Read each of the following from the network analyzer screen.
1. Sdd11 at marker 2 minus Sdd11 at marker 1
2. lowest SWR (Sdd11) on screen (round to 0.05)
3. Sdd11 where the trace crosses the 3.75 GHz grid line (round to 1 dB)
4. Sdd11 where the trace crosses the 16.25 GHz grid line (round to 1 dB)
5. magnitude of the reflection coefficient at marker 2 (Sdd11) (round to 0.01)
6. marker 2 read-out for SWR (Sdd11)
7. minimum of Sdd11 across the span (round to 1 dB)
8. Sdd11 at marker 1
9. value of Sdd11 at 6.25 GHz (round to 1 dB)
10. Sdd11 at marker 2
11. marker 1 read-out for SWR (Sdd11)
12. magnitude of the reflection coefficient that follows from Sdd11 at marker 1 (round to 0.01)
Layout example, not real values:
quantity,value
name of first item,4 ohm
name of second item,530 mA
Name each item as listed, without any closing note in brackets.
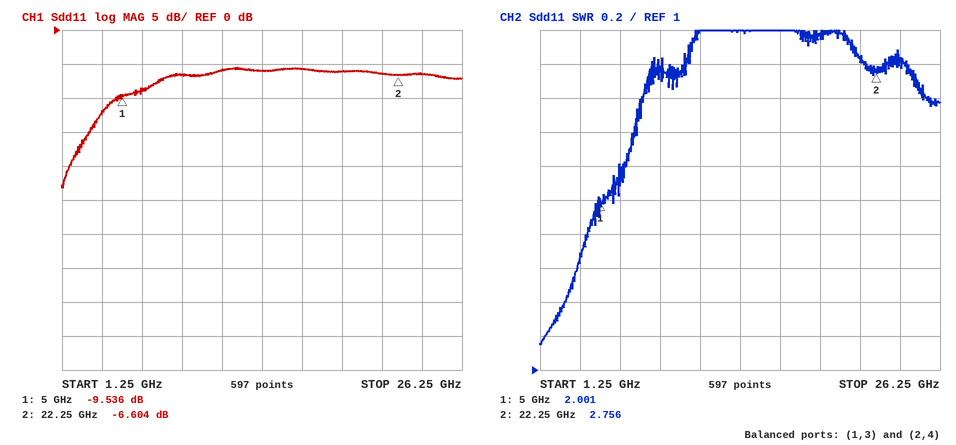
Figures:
quantity,value
Sdd11 at marker 2 minus Sdd11 at marker 1,2.932 dB
lowest SWR (Sdd11) on screen,1.15
Sdd11 where the trace crosses the 3.75 GHz grid line,-12 dB
Sdd11 where the trace crosses the 16.25 GHz grid line,-6 dB
magnitude of the reflection coefficient at marker 2 (Sdd11),0.47
marker 2 read-out for SWR,2.756
minimum of Sdd11 across the span,-23 dB
Sdd11 at marker 1,-9.536 dB
value of Sdd11 at 6.25 GHz,-9 dB
Sdd11 at marker 2,-6.604 dB
marker 1 read-out for SWR,2.001
magnitude of the reflection coefficient that follows from Sdd11 at marker 1,0.33
